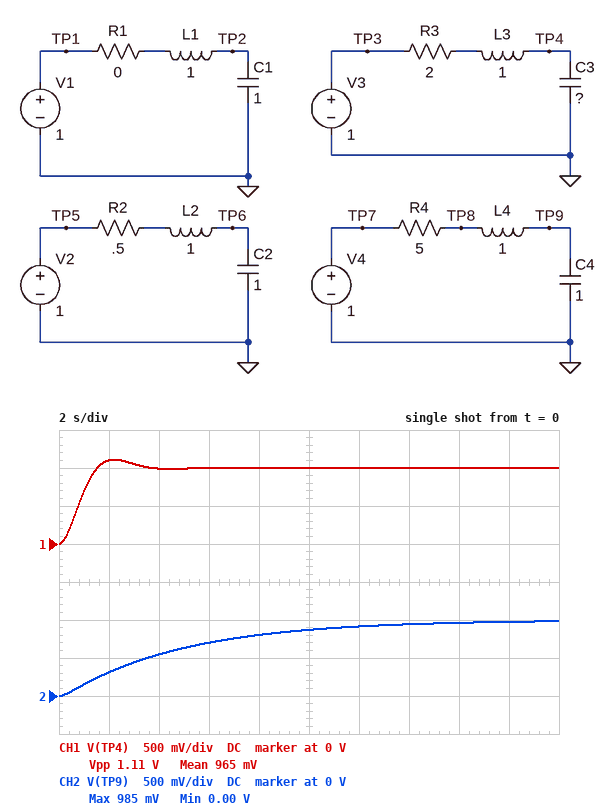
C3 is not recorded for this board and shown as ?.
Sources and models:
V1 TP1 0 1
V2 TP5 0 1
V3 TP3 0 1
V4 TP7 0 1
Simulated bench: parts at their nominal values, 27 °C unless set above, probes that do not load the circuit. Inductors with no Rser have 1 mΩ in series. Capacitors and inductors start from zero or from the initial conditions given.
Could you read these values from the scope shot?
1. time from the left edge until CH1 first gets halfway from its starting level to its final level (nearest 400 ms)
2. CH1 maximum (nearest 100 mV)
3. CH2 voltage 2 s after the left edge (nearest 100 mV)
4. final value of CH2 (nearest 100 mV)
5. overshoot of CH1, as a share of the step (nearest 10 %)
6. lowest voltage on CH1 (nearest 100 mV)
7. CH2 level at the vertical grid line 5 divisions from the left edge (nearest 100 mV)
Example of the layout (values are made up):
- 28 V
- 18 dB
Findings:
- 800 ms
- 1.1 V
- 300 mV
- 1.0 V
- 10 %
- 0 V
- 900 mV
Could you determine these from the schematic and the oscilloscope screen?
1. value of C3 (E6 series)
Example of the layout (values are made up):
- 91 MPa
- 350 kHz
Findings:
- 330 mF
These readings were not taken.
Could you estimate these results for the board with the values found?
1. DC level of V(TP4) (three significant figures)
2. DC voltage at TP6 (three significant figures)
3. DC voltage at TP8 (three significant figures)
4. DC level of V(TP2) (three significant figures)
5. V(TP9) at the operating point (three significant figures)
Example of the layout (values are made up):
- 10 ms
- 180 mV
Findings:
- 1.00 V
- 1.00 V
- 1.00 V
- 1.00 V
- 1.00 V
